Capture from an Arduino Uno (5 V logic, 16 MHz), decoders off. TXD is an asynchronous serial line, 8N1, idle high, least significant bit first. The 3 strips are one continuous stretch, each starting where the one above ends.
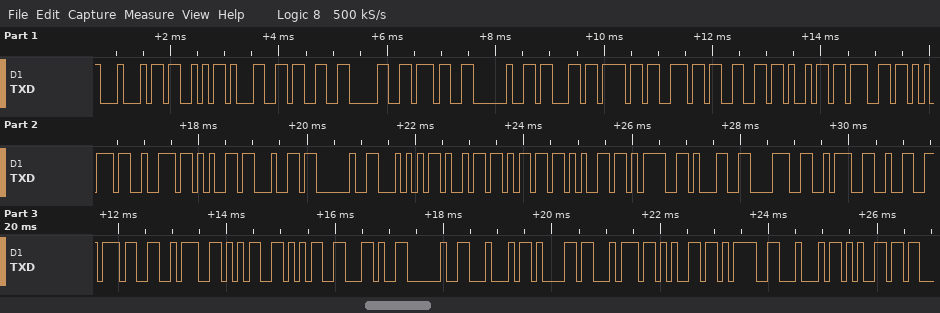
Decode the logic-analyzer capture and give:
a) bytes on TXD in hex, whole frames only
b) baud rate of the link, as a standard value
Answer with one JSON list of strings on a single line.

["44 53 31 33 30 37 20 63 6F 6E 66 69 67 75 72 65 64 20 54 69 6D 65 3D 31 38 3A 32 37 3A 35 35 2C 20 44 61 74 65 3D 44 65", "9600 baud"]
